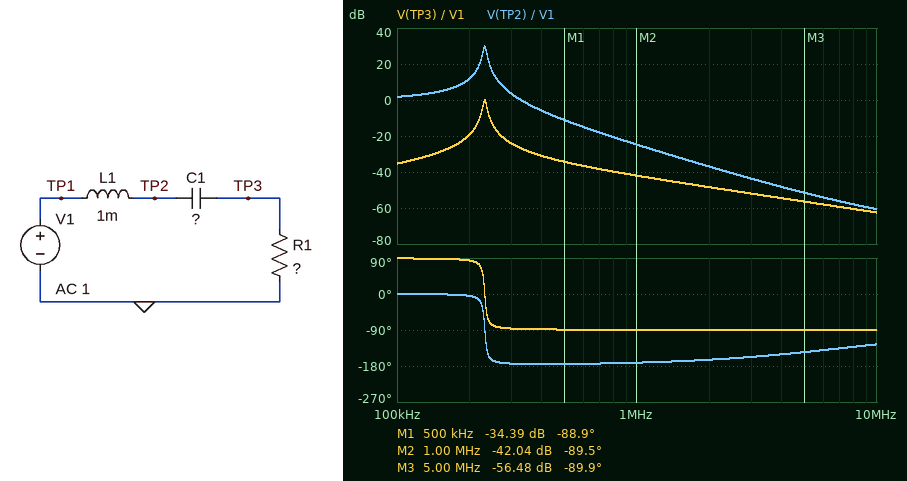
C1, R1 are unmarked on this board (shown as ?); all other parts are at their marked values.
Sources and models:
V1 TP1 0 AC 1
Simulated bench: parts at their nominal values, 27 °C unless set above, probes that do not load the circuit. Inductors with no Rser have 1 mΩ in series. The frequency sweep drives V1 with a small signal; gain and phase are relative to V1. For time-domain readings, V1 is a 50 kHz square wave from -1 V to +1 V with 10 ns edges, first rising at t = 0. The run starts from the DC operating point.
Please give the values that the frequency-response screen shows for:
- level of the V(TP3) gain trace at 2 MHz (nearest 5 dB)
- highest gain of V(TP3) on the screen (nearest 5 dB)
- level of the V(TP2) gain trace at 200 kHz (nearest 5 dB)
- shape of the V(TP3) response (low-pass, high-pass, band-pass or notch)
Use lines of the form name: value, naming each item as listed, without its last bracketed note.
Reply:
level of the V(TP3) gain trace at 2 MHz: -50 dB
highest gain of V(TP3) on the screen: 0 dB
level of the V(TP2) gain trace at 200 kHz: 10 dB
shape of the V(TP3) response: band-pass
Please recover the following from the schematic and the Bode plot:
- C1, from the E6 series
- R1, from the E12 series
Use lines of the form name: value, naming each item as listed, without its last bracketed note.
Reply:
C1, from the E6 series: 470 pF
R1, from the E12 series: 47 Ω
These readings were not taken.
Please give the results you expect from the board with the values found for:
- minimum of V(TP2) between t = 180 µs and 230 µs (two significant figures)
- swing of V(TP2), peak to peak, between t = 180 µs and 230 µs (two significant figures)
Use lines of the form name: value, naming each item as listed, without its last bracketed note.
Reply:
minimum of V(TP2) between t = 180 µs and 230 µs: -2.9 V
swing of V(TP2), peak to peak, between t = 180 µs and 230 µs: 5.9 V
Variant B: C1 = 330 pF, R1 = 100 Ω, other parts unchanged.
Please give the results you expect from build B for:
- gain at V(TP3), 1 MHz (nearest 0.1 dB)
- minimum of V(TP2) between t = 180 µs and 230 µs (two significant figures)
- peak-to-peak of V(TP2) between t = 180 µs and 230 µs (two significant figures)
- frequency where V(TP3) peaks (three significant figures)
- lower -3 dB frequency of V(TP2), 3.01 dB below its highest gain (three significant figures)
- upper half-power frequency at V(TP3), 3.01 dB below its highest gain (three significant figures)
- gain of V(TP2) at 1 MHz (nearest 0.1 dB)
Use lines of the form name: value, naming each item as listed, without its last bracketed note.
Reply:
gain at V(TP3), 1 MHz: -35.3 dB
minimum of V(TP2) between t = 180 µs and 230 µs: -2.5 V
peak-to-peak of V(TP2) between t = 180 µs and 230 µs: 5.0 V
frequency where V(TP3) peaks: 277 kHz
lower -3 dB frequency of V(TP2), 3.01 dB below its highest gain: 269 kHz
upper half-power frequency at V(TP3), 3.01 dB below its highest gain: 285 kHz
gain of V(TP2) at 1 MHz: -21.4 dB
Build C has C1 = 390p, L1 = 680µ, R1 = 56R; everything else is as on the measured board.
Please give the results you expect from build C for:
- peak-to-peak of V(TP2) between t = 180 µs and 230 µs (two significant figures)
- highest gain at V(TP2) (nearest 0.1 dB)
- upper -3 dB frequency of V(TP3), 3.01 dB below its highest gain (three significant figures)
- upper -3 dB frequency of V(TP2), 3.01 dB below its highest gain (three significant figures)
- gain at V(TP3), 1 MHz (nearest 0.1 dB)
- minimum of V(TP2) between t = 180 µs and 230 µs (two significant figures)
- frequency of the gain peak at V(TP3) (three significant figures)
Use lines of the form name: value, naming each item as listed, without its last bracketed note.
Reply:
peak-to-peak of V(TP2) between t = 180 µs and 230 µs: 4.3 V
highest gain at V(TP2): 27.5 dB
upper -3 dB frequency of V(TP3), 3.01 dB below its highest gain: 316 kHz
upper -3 dB frequency of V(TP2), 3.01 dB below its highest gain: 315 kHz
gain at V(TP3), 1 MHz: -36.8 dB
minimum of V(TP2) between t = 180 µs and 230 µs: -2.2 V
frequency of the gain peak at V(TP3): 309 kHz
